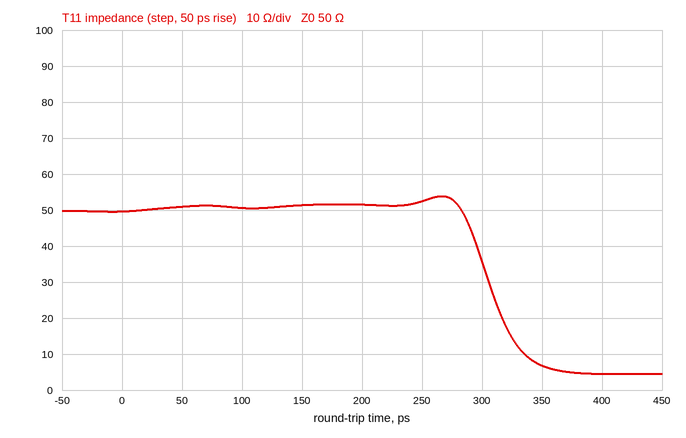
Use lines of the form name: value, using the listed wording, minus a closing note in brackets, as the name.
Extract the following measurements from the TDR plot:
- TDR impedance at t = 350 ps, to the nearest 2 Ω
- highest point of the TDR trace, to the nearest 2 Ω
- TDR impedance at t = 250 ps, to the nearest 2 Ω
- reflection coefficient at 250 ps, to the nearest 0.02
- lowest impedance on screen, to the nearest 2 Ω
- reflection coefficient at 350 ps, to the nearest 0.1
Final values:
TDR impedance at t = 350 ps, to the nearest 2 Ω: 6 Ω
highest point of the TDR trace, to the nearest 2 Ω: 54 Ω
TDR impedance at t = 250 ps, to the nearest 2 Ω: 52 Ω
reflection coefficient at 250 ps, to the nearest 0.02: +0.02
lowest impedance on screen, to the nearest 2 Ω: 4 Ω
reflection coefficient at 350 ps, to the nearest 0.1: -0.8
